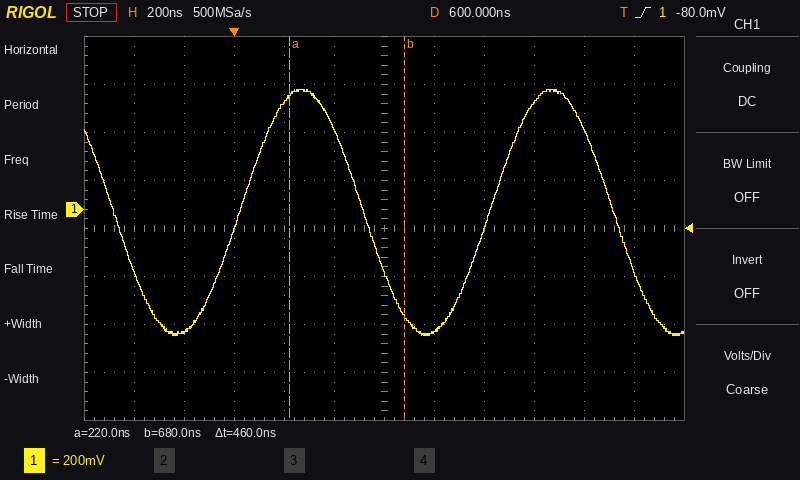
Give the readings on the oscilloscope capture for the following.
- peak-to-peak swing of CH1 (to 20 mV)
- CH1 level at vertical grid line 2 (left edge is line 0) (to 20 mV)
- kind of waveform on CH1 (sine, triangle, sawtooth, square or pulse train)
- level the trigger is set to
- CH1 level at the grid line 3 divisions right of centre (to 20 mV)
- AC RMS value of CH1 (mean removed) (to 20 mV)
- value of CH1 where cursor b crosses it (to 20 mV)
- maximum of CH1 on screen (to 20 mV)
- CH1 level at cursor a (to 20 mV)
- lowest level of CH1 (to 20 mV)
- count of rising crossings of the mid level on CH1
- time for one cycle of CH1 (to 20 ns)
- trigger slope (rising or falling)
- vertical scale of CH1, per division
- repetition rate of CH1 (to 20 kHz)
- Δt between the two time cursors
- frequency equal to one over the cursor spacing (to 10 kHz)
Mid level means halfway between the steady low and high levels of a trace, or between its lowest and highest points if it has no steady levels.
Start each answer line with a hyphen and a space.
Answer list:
- 1.02 V
- -500 mV
- sine
- -80.0 mV
- 440 mV
- 360 mV
- -440 mV
- 500 mV
- 480 mV
- -520 mV
- 2
- 1.00 µs
- rising
- 200 mV
- 1.00 MHz
- 460 ns
- 2.17 MHz
